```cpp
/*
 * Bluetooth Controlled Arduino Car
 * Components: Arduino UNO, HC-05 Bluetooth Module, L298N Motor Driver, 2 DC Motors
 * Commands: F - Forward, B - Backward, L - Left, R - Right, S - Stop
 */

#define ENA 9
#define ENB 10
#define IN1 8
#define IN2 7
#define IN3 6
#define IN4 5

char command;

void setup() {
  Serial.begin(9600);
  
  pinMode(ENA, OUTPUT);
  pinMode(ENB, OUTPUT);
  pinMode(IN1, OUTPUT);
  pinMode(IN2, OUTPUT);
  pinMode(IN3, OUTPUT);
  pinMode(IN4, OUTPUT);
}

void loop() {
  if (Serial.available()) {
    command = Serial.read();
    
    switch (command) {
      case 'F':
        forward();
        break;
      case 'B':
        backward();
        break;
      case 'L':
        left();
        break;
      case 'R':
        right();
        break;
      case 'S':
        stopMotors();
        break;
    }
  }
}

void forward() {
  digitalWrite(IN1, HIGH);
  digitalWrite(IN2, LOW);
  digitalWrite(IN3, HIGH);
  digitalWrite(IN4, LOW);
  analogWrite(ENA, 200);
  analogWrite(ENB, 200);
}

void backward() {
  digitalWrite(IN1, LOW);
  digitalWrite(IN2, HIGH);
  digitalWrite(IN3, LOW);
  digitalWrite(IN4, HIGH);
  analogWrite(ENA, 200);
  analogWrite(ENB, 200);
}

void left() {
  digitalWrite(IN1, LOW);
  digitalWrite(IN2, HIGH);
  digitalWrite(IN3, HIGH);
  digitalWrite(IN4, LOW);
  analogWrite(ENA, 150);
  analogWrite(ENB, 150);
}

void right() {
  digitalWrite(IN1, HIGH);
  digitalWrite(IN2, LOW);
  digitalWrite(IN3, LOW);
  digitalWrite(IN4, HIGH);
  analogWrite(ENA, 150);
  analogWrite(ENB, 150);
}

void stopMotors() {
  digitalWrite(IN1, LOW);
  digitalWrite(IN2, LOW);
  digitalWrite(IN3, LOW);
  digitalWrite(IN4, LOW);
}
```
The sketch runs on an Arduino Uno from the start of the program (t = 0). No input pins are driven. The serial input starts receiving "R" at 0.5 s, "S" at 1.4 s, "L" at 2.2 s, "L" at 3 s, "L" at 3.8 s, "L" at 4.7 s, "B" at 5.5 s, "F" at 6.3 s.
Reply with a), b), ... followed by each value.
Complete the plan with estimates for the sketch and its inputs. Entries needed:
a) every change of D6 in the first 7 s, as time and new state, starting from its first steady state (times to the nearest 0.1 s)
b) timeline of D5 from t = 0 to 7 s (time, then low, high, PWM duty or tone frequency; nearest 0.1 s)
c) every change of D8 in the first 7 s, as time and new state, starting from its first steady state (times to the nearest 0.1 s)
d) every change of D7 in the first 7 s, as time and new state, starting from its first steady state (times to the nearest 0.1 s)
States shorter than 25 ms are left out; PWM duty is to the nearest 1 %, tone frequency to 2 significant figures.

a) 0 s low; 2.2 s high; 5.5 s low; 6.3 s high
b) 0 s low; 0.5 s high; 1.4 s low; 5.5 s high; 6.3 s low
c) 0 s low; 0.5 s high; 1.4 s low; 6.3 s high
d) 0 s low; 2.2 s high; 6.3 s low
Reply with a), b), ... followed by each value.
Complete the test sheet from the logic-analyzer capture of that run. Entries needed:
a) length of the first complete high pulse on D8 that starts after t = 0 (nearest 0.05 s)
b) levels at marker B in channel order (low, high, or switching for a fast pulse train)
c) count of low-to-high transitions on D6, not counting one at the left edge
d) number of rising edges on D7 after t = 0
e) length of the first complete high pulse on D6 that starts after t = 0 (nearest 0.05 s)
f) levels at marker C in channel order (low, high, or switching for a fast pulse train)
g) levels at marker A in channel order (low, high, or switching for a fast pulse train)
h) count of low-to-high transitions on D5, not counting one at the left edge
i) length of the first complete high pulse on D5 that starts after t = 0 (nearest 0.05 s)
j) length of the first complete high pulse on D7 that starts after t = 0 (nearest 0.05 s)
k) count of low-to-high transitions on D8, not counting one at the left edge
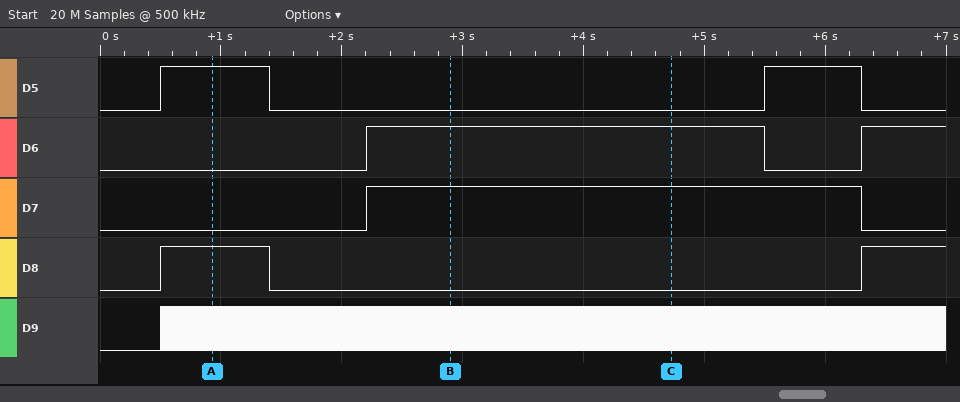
a) 0.90 s
b) D5 low, D6 high, D7 high, D8 low, D9 switching
c) 2
d) 1
e) 3.30 s
f) D5 low, D6 high, D7 high, D8 low, D9 switching
g) D5 high, D6 low, D7 low, D8 high, D9 switching
h) 2
i) 0.90 s
j) 4.10 s
k) 2
